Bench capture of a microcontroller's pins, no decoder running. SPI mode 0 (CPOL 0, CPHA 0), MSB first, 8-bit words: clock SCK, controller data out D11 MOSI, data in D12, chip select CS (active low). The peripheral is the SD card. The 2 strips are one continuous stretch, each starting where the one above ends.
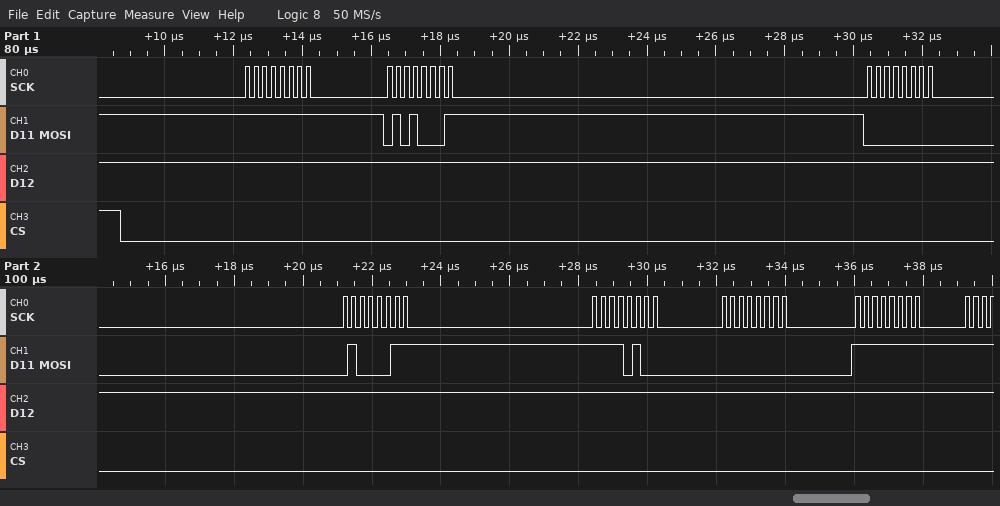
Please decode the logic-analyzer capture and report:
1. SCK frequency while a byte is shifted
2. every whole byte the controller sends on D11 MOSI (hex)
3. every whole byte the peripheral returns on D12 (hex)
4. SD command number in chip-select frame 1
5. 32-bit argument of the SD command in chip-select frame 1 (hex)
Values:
4 MHz
FF 51 00 43 F4 00 FF
FF FF FF FF FF FF FF
CMD17
0x0043F400
